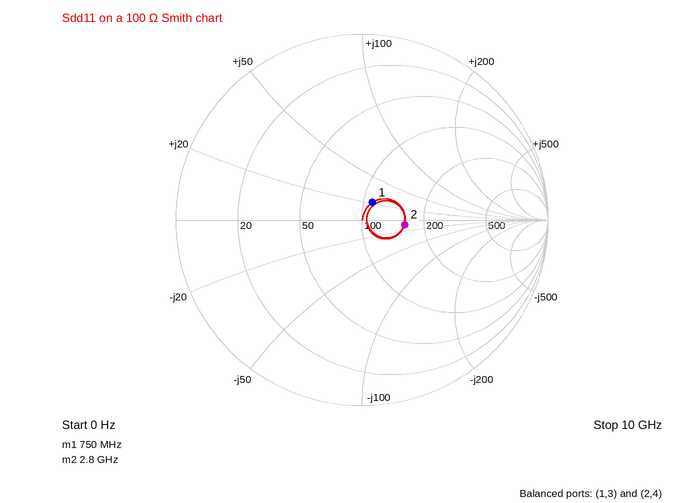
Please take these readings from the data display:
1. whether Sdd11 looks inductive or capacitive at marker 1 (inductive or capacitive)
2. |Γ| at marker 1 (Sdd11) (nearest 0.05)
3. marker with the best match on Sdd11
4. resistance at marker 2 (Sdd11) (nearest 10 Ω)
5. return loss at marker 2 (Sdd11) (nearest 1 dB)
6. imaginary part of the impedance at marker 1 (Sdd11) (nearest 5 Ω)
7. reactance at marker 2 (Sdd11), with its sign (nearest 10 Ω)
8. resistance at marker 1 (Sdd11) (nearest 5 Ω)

inductive
0.10
marker 1
160 Ω
13 dB
+20 Ω
-10 Ω
110 Ω
